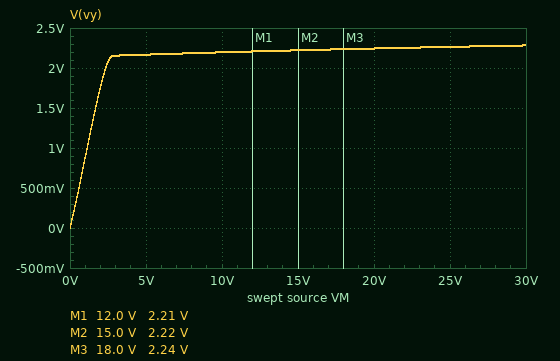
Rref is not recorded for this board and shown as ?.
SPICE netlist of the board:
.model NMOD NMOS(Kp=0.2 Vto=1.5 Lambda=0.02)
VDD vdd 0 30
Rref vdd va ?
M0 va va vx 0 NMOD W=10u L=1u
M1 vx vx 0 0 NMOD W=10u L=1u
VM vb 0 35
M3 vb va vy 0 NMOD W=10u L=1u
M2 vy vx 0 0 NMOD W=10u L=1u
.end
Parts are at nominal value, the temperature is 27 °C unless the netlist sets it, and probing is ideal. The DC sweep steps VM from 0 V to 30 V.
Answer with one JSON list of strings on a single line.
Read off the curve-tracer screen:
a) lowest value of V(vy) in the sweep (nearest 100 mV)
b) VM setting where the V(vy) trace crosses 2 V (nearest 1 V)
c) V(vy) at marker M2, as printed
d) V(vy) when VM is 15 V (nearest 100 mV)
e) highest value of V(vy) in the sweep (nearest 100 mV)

["0 V", "2 V", "2.22 V", "2.2 V", "2.3 V"]
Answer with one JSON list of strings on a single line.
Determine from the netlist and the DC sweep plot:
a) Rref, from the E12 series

["56 Ω"]
